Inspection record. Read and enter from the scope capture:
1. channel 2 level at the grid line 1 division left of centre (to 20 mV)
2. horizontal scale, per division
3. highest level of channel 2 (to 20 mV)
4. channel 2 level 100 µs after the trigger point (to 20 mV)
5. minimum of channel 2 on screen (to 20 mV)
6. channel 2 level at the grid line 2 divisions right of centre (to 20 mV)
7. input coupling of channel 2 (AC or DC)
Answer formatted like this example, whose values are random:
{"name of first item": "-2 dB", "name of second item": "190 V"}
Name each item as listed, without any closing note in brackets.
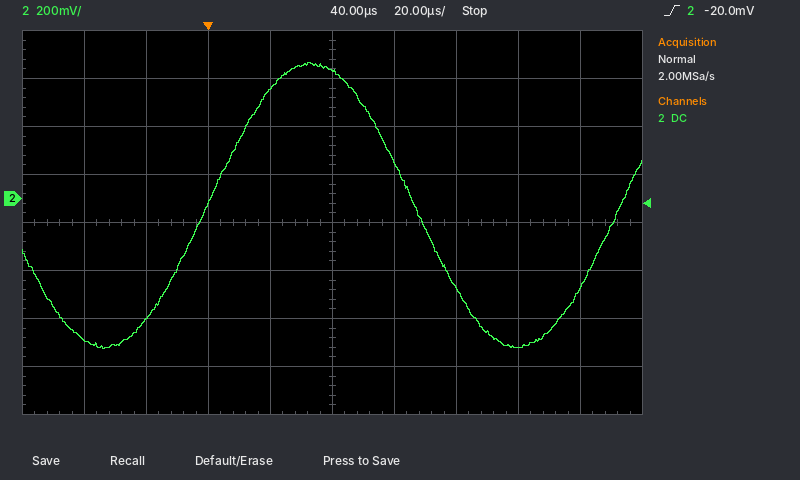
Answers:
{"channel 2 level at the grid line 1 division left of centre": "460 mV", "horizontal scale, per division": "20 µs", "highest level of channel 2": "560 mV", "channel 2 level 100 µs after the trigger point": "-620 mV", "minimum of channel 2 on screen": "-620 mV", "channel 2 level at the grid line 2 divisions right of centre": "-380 mV", "input coupling of channel 2": "DC"}
